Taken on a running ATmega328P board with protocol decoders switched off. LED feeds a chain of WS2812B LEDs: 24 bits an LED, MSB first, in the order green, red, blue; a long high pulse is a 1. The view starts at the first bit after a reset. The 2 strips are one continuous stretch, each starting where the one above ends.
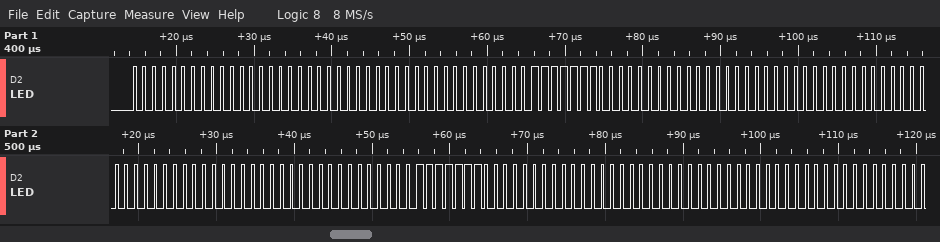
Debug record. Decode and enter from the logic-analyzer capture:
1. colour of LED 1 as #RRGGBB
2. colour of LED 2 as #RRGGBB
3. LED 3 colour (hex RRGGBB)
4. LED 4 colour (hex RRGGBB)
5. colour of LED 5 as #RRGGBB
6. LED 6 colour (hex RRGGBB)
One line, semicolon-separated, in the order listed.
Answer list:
#000000; #00007F; #000000; #000000; #00007F; #000000
